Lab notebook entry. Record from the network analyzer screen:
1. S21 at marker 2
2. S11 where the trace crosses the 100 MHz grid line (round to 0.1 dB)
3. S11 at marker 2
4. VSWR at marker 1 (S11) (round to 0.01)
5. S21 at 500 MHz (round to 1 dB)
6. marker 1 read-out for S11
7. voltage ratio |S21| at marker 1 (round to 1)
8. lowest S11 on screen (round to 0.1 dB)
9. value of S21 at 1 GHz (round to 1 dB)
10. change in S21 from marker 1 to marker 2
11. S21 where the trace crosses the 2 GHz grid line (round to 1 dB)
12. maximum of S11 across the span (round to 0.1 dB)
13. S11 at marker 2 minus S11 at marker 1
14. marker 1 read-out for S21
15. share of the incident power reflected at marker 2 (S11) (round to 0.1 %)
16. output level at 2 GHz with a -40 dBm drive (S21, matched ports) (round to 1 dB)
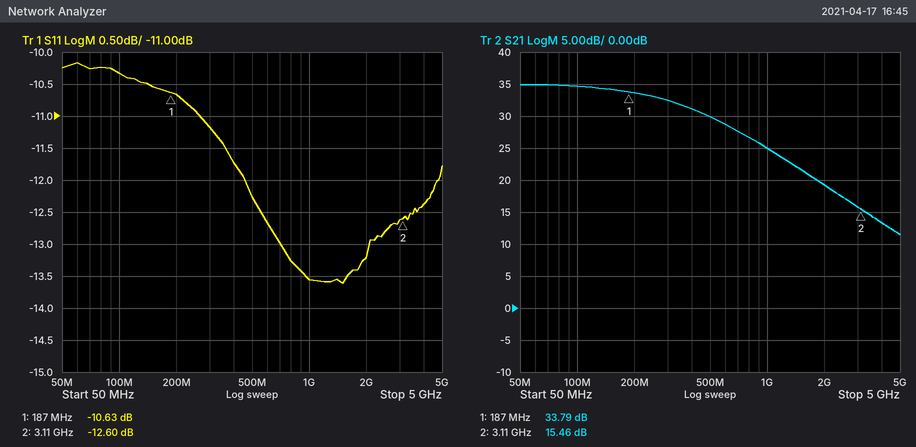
15.46 dB
-10.3 dB
-12.60 dB
1.83
30 dB
-10.63 dB
49
-13.6 dB
25 dB
-18.33 dB
19 dB
-10.2 dB
-1.97 dB
33.79 dB
5.5 %
-21 dBm
